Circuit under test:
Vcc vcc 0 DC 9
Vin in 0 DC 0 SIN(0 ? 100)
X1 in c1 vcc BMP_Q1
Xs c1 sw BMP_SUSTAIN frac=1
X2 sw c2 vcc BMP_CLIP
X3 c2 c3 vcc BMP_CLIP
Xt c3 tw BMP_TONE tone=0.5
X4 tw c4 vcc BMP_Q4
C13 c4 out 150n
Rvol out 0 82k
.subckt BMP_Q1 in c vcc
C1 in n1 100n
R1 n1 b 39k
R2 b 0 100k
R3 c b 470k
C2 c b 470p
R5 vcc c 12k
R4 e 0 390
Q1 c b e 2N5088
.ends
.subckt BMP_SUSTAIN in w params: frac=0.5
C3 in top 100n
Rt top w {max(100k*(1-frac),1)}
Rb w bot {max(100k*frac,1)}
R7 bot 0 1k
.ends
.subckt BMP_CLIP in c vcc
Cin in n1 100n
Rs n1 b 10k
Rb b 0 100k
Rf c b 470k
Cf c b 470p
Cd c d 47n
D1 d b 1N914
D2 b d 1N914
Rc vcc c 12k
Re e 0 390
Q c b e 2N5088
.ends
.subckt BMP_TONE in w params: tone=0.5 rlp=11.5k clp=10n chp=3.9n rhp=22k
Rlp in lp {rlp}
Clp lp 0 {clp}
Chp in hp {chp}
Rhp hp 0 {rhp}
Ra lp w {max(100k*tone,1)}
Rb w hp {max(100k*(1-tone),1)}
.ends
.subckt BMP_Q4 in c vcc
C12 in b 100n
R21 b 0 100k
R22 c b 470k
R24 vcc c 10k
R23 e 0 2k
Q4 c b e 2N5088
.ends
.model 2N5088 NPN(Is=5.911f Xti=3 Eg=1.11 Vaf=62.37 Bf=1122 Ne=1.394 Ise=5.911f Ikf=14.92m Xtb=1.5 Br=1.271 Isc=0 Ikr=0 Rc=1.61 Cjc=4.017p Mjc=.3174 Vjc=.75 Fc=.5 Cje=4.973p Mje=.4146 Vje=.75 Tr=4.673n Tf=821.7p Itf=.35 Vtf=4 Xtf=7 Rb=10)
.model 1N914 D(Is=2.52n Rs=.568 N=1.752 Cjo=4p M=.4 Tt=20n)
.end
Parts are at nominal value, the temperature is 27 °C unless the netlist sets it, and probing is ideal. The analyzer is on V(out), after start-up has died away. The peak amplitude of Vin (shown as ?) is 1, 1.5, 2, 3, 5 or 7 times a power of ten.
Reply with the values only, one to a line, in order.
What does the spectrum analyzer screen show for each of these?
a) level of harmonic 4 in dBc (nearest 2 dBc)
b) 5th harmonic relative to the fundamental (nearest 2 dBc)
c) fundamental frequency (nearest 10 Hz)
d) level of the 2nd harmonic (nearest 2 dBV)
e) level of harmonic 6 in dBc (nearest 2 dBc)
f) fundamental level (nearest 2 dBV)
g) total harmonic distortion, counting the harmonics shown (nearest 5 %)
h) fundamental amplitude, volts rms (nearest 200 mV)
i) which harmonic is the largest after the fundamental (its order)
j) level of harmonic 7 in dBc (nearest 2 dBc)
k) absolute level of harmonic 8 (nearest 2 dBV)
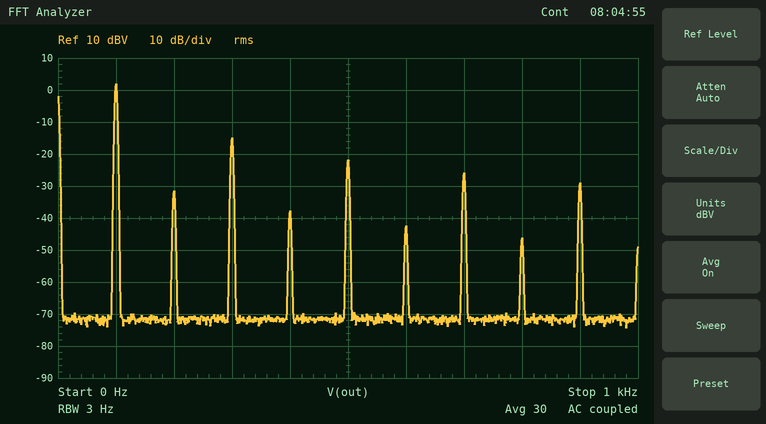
-40 dBc
-24 dBc
100 Hz
-32 dBV
-44 dBc
2 dBV
15 %
1.2 V
3
-28 dBc
-46 dBV
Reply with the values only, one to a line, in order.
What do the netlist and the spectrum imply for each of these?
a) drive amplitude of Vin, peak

150 mV
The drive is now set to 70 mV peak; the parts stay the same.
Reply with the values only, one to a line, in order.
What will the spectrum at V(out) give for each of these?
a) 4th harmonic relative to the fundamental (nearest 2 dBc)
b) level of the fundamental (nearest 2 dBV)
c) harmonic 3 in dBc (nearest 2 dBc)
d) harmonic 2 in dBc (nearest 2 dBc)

-52 dBc
0 dBV
-16 dBc
-42 dBc
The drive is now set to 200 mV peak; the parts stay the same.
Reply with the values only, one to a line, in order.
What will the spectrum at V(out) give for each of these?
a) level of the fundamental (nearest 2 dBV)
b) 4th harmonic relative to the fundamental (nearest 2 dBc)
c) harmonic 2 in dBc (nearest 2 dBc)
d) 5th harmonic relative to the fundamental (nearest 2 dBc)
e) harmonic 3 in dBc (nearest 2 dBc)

4 dBV
-30 dBc
-26 dBc
-28 dBc
-20 dBc
